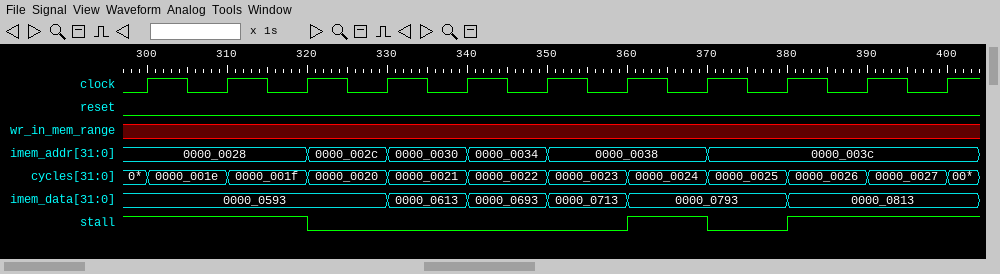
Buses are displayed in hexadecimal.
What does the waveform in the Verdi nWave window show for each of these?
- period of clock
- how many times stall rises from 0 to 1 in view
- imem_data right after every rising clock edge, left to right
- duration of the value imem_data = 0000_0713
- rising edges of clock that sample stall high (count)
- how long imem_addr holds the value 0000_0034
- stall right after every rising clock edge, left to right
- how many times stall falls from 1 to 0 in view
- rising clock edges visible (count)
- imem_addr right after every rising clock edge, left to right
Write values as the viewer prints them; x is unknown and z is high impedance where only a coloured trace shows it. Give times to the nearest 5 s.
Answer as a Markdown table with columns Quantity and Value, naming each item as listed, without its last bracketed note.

| Quantity | Value |
|---|---|
| period of clock | 10 s |
| how many times stall rises from 0 to 1 in view | 2 |
| imem_data right after every rising clock edge, left to right | 0000_0593, 0000_0593, 0000_0593, 0000_0613, 0000_0693, 0000_0713, 0000_0793, 0000_0793, 0000_0813, 0000_0813, 0000_0813 |
| duration of the value imem_data = 0000_0713 | 10 s |
| rising edges of clock that sample stall high | 6 |
| how long imem_addr holds the value 0000_0034 | 10 s |
| stall right after every rising clock edge, left to right | 1 1 0 0 0 0 1 0 1 1 1 |
| how many times stall falls from 1 to 0 in view | 2 |
| rising clock edges visible | 11 |
| imem_addr right after every rising clock edge, left to right | 0000_0028, 0000_0028, 0000_002c, 0000_0030, 0000_0034, 0000_0038, 0000_0038, 0000_003c, 0000_003c, 0000_003c, 0000_003c |
